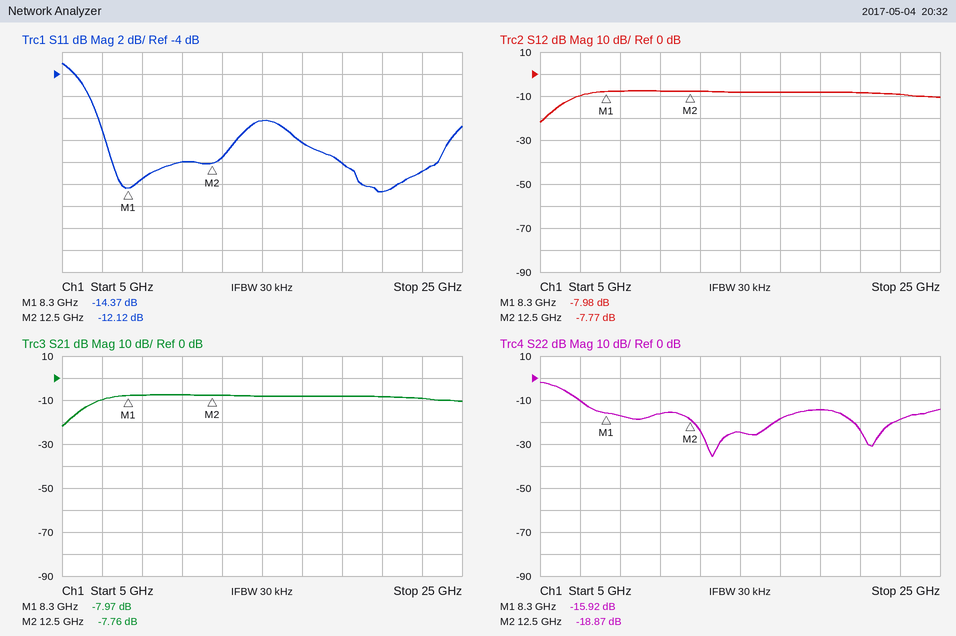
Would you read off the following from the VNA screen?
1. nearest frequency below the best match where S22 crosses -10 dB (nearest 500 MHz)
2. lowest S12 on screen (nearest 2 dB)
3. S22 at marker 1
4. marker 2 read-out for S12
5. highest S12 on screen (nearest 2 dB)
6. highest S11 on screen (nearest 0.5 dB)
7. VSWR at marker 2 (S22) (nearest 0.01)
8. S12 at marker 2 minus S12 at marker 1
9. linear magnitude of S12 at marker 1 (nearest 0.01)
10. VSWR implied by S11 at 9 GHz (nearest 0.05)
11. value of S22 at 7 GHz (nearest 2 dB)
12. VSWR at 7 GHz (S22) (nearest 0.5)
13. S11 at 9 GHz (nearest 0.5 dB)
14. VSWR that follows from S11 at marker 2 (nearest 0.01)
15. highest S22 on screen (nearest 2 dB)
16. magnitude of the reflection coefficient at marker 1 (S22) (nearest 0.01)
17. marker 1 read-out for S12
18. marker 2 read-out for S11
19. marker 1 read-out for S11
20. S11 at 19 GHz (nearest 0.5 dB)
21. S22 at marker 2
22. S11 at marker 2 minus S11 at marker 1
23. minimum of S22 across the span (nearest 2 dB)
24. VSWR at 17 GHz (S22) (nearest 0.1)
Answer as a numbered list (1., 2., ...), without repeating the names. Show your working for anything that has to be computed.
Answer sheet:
1. 7.0 GHz
2. -22 dB
3. -15.92 dB
4. -7.77 dB
5. -8 dB
6. -3.0 dB
7. (1 + 0.1139)/(1 − 0.1139) ≈ 1.26
8. -7.77 − (-7.98) = 0.21 dB
9. 10^(-7.98/20) ≈ 0.40
10. |Γ| = 10^(-13.5/20) = 0.2113; VSWR = (1 + 0.2113)/(1 − 0.2113) ≈ 1.54, so 1.55 to the nearest 0.05
11. -10 dB
12. |Γ| = 10^(-10/20) = 0.3162; VSWR = (1 + 0.3162)/(1 − 0.3162) ≈ 1.92, so 2.0 to the nearest 0.5
13. -13.5 dB
14. (1 + 0.2477)/(1 − 0.2477) ≈ 1.66
15. -2 dB
16. 10^(-15.92/20) ≈ 0.16
17. -7.98 dB
18. -12.12 dB
19. -14.37 dB
20. -12.0 dB
21. -18.87 dB
22. -12.12 − (-14.37) = 2.25 dB
23. -36 dB
24. |Γ| = 10^(-18/20) = 0.1259; VSWR = (1 + 0.1259)/(1 − 0.1259) ≈ 1.3
